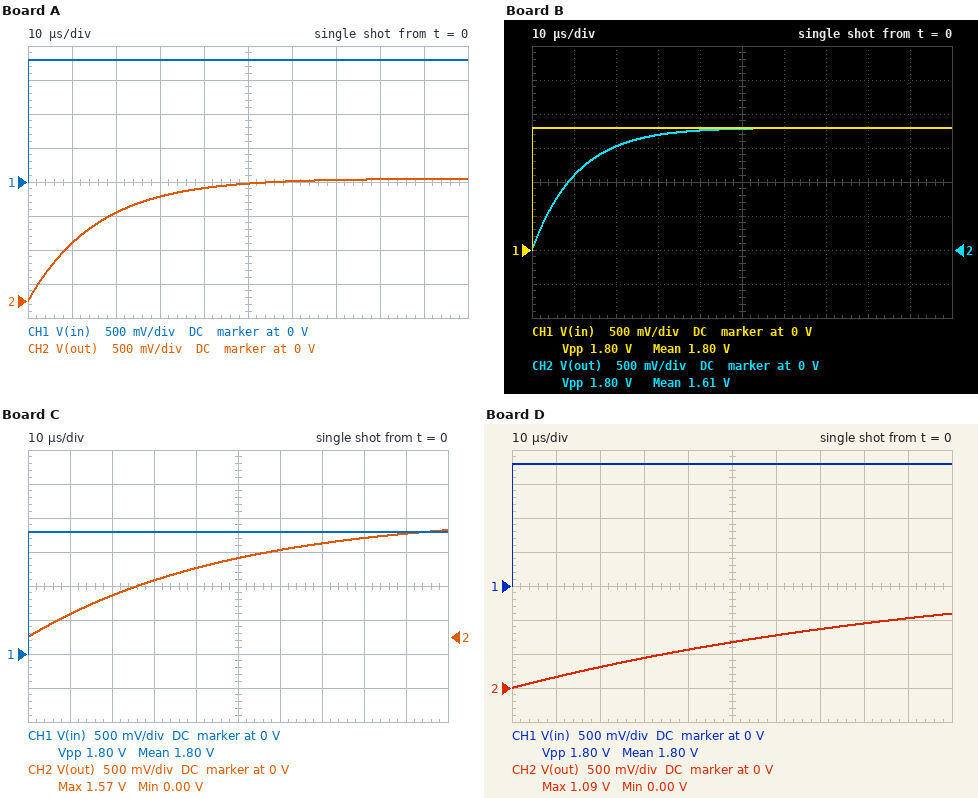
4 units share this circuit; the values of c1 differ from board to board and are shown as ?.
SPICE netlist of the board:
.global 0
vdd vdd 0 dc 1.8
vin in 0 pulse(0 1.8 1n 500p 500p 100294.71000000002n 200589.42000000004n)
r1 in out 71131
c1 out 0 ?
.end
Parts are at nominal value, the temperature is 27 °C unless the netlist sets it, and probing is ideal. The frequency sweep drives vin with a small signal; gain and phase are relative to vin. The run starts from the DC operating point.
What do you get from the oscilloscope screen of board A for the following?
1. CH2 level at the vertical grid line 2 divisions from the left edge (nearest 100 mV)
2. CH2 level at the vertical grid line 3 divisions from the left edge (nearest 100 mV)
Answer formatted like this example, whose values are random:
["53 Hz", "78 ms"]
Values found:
["1.3 V", "1.5 V"]
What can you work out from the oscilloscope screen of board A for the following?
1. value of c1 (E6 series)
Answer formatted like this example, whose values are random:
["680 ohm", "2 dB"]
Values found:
["220 pF"]
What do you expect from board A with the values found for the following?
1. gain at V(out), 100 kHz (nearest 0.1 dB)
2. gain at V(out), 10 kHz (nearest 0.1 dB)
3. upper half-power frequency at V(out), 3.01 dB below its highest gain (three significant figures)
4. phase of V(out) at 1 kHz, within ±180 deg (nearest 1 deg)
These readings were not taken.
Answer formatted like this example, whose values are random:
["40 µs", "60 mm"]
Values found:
["-19.9 dB", "-2.9 dB", "10.2 kHz", "-6 deg"]
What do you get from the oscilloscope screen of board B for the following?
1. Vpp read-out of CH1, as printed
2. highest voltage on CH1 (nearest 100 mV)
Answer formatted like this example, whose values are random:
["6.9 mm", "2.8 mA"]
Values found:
["1.80 V", "1.8 V"]
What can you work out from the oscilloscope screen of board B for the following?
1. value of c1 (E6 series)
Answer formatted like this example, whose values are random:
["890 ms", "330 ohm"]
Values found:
["150 pF"]
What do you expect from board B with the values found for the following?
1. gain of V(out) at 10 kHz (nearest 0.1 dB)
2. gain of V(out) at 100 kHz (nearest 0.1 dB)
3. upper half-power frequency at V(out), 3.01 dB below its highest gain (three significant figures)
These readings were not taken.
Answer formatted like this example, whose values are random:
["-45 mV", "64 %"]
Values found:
["-1.6 dB", "-16.6 dB", "14.9 kHz"]
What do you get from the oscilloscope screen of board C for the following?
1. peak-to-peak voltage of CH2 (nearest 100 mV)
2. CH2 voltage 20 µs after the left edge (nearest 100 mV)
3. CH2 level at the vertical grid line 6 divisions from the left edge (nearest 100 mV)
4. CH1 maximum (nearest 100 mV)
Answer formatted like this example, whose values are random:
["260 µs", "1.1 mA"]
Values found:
["1.6 V", "600 mV", "1.3 V", "1.8 V"]
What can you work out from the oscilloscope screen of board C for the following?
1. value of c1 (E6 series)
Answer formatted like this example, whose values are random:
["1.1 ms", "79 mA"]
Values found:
["680 pF"]
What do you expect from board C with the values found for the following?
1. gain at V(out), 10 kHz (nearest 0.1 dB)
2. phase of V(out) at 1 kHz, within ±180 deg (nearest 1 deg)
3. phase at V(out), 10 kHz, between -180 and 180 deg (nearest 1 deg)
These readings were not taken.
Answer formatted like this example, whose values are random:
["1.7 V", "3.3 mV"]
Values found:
["-10.1 dB", "-17 deg", "-72 deg"]
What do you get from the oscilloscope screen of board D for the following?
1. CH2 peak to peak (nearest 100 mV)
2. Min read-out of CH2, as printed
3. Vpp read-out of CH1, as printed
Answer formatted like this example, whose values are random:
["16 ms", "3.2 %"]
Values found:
["1.1 V", "0.00 V", "1.80 V"]
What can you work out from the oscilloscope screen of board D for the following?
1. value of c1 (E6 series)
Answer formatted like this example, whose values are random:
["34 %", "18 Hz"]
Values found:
["1.5 nF"]
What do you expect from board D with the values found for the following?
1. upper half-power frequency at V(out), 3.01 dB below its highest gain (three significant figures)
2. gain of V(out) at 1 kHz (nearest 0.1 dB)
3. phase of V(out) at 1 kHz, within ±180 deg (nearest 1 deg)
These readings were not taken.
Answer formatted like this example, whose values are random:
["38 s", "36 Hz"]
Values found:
["1.49 kHz", "-1.6 dB", "-34 deg"]
